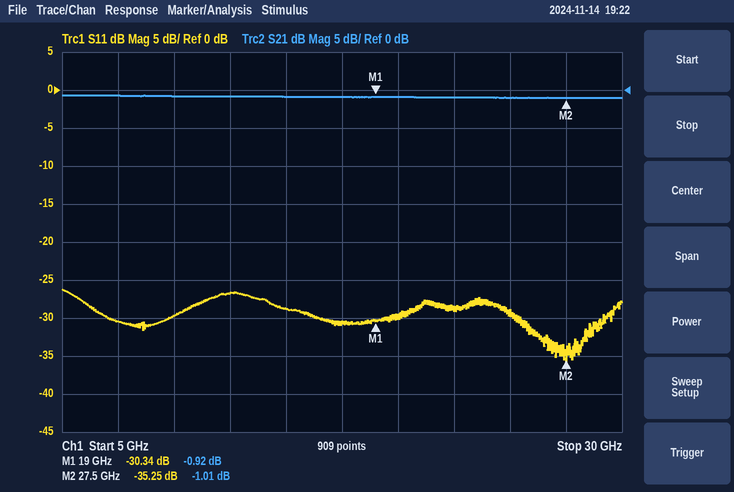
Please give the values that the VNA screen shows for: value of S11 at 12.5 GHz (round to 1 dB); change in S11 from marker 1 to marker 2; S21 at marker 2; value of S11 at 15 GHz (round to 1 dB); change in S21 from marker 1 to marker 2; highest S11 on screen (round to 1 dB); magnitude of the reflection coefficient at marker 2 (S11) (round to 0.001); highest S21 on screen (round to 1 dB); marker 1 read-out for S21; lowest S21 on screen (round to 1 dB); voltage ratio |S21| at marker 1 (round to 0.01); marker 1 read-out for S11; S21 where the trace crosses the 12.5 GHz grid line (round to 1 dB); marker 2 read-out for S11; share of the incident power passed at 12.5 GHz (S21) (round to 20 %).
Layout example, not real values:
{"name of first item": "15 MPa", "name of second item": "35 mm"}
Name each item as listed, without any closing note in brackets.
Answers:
{"value of S11 at 12.5 GHz": "-27 dB", "change in S11 from marker 1 to marker 2": "-4.91 dB", "S21 at marker 2": "-1.01 dB", "value of S11 at 15 GHz": "-29 dB", "change in S21 from marker 1 to marker 2": "-0.09 dB", "highest S11 on screen": "-26 dB", "magnitude of the reflection coefficient at marker 2 (S11)": "0.017", "highest S21 on screen": "-1 dB", "marker 1 read-out for S21": "-0.92 dB", "lowest S21 on screen": "-1 dB", "voltage ratio |S21| at marker 1": "0.90", "marker 1 read-out for S11": "-30.34 dB", "S21 where the trace crosses the 12.5 GHz grid line": "-1 dB", "marker 2 read-out for S11": "-35.25 dB", "share of the incident power passed at 12.5 GHz (S21)": "80 %"}
